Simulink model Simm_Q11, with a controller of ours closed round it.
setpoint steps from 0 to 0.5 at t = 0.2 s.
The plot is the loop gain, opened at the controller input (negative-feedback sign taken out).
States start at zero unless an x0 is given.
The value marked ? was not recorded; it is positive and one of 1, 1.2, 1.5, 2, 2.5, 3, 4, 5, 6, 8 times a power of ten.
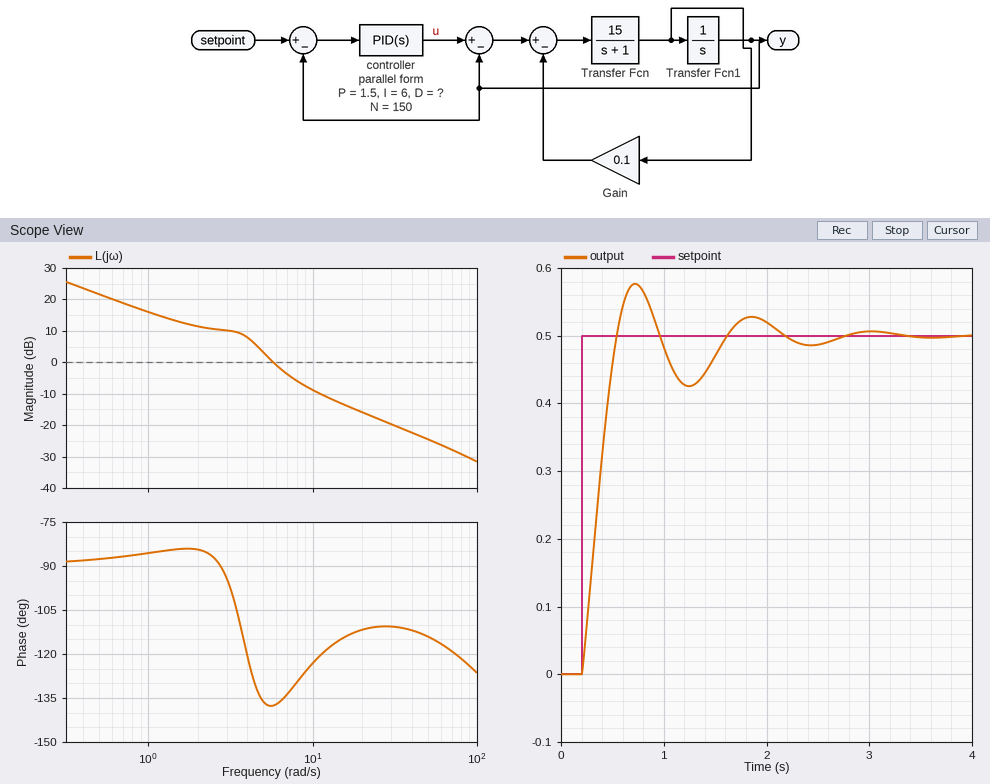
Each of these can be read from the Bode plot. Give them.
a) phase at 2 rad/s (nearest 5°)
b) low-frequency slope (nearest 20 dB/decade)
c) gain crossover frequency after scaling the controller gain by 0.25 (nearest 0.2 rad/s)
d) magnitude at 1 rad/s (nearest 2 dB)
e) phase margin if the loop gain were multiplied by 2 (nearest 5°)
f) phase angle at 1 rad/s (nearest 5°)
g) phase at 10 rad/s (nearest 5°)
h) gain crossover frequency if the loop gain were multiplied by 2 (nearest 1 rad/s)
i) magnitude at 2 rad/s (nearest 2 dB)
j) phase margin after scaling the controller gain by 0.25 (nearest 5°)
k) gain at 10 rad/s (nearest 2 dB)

-85°
-20 dB/decade
1.8 rad/s
16 dB
50°
-85°
-125°
8 rad/s
12 dB
95°
-8 dB
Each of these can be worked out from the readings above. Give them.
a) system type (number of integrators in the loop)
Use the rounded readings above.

1
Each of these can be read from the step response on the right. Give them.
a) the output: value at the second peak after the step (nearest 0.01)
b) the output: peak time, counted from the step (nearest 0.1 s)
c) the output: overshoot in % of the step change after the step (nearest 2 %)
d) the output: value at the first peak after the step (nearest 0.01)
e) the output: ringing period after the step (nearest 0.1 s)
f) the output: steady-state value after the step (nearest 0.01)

0.53
0.5 s
16 %
0.58
1.1 s
0.50
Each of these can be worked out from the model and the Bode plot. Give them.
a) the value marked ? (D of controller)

0.2
